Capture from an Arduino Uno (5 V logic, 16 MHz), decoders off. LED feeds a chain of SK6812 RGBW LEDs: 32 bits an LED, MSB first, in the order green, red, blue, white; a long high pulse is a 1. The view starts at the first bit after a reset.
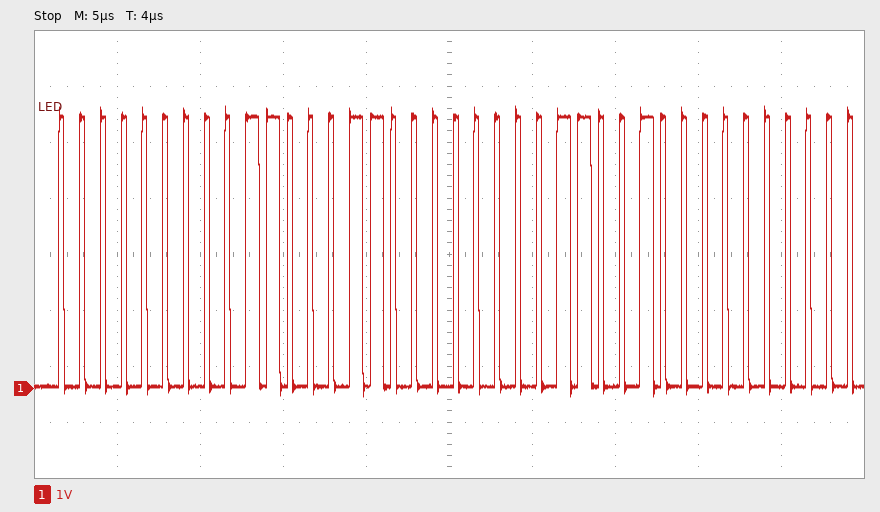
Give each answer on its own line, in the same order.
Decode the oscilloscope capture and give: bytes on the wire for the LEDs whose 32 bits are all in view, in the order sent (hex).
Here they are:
00 63 00 C8
